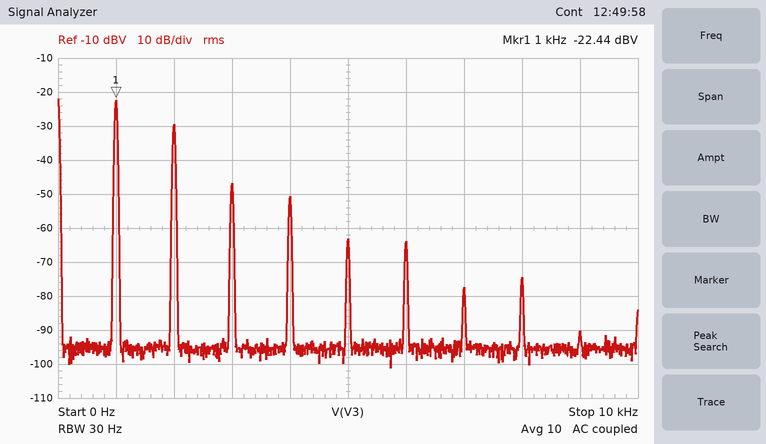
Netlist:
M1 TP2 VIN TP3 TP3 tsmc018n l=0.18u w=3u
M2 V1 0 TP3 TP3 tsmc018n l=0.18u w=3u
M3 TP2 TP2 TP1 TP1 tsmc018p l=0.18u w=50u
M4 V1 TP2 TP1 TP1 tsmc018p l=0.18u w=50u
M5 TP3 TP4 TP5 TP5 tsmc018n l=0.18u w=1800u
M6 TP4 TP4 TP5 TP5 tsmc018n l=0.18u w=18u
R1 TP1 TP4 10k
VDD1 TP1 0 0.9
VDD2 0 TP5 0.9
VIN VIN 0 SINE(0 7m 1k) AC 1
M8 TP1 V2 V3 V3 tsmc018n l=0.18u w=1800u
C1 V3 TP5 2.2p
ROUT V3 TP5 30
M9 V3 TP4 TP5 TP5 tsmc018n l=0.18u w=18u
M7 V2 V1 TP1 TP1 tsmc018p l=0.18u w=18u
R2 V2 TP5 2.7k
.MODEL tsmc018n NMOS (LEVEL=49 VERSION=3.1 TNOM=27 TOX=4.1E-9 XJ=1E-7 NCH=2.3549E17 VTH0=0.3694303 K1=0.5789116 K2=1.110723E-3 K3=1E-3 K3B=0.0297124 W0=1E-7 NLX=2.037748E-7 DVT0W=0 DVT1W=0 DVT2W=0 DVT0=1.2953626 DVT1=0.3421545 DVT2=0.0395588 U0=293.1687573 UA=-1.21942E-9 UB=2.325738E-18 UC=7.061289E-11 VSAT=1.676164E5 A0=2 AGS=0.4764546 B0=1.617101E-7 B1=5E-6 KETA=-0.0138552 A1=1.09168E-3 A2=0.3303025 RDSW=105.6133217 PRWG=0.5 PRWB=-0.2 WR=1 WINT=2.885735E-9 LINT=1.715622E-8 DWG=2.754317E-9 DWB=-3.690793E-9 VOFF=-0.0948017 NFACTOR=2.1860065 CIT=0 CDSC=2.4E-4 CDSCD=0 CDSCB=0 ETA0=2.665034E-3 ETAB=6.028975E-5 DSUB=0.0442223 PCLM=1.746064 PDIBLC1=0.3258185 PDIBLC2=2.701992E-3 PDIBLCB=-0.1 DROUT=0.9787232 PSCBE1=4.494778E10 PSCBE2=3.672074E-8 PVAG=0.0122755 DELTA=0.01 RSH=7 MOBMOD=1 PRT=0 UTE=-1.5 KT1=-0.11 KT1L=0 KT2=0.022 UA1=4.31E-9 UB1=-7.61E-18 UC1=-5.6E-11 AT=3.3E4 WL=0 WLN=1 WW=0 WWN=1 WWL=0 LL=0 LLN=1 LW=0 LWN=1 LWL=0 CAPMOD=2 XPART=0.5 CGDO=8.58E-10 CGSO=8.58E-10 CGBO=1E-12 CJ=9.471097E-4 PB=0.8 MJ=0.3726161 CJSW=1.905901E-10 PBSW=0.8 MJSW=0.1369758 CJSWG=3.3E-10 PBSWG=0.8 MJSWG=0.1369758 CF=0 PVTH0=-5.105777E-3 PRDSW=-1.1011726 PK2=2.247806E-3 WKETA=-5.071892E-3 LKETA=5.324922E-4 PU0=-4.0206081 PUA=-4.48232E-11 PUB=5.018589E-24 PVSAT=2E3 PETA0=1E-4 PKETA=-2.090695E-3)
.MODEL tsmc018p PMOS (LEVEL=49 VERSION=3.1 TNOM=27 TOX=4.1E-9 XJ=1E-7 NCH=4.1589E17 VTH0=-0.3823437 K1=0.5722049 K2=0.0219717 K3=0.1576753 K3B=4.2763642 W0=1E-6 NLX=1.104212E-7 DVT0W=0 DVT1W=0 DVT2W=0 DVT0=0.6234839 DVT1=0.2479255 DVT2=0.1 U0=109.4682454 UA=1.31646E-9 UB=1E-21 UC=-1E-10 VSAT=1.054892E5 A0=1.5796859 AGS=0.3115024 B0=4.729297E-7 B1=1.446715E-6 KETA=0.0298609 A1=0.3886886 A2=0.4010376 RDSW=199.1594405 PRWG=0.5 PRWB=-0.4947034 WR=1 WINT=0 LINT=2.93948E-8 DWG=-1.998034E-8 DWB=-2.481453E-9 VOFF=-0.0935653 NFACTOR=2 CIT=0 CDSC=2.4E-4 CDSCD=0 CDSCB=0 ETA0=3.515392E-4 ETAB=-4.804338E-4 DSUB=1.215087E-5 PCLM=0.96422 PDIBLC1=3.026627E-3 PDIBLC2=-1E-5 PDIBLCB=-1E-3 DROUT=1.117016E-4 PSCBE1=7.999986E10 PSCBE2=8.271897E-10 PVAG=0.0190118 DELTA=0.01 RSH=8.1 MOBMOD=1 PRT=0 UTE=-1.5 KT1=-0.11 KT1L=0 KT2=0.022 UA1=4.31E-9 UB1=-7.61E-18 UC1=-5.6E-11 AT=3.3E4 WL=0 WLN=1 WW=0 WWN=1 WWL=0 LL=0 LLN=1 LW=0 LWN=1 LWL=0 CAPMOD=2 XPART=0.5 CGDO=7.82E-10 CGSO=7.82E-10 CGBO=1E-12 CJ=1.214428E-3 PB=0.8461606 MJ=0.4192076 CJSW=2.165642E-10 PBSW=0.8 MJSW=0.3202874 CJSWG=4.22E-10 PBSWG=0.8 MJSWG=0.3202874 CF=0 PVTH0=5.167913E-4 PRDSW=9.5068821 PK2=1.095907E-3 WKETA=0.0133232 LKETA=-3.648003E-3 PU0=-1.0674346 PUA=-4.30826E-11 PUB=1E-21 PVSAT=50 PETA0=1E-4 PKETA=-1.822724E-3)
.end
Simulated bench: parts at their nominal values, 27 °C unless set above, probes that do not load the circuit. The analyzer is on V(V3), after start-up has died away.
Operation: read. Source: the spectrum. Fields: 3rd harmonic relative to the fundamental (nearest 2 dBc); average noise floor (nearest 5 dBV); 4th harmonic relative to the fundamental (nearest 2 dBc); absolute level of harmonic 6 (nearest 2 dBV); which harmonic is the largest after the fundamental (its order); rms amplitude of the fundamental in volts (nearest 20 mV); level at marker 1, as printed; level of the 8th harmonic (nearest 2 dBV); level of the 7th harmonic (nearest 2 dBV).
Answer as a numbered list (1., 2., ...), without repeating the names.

1. -24 dBc
2. -95 dBV
3. -28 dBc
4. -64 dBV
5. 2
6. 80 mV
7. -22.44 dBV
8. -74 dBV
9. -78 dBV
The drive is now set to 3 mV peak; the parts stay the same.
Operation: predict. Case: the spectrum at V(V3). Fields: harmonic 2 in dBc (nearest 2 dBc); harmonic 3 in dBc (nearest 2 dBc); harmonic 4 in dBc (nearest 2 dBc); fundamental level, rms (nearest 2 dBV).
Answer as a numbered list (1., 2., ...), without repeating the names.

1. -10 dBc
2. -32 dBc
3. -38 dBc
4. -32 dBV
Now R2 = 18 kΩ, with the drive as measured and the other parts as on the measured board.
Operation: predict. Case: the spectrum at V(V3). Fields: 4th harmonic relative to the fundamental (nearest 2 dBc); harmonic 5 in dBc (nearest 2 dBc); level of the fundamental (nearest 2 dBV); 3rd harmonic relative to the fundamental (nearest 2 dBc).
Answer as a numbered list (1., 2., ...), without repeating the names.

1. -26 dBc
2. -26 dBc
3. -14 dBV
4. -20 dBc
